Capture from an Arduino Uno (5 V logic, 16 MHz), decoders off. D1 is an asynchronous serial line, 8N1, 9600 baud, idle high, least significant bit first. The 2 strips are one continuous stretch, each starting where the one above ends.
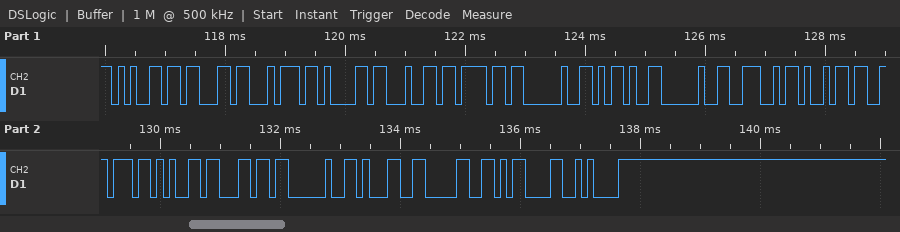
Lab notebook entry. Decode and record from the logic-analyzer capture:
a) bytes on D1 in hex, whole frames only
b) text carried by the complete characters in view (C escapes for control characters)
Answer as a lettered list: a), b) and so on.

a) 0x65 0x63 0x74 0x61 0x64 0x6F 0x20 0x2D 0x20 0x4E 0x69 0x76 0x65 0x6C 0x20 0x31 0x30 0x0D 0x0A
b) "ectado - Nivel 10\r\n"
